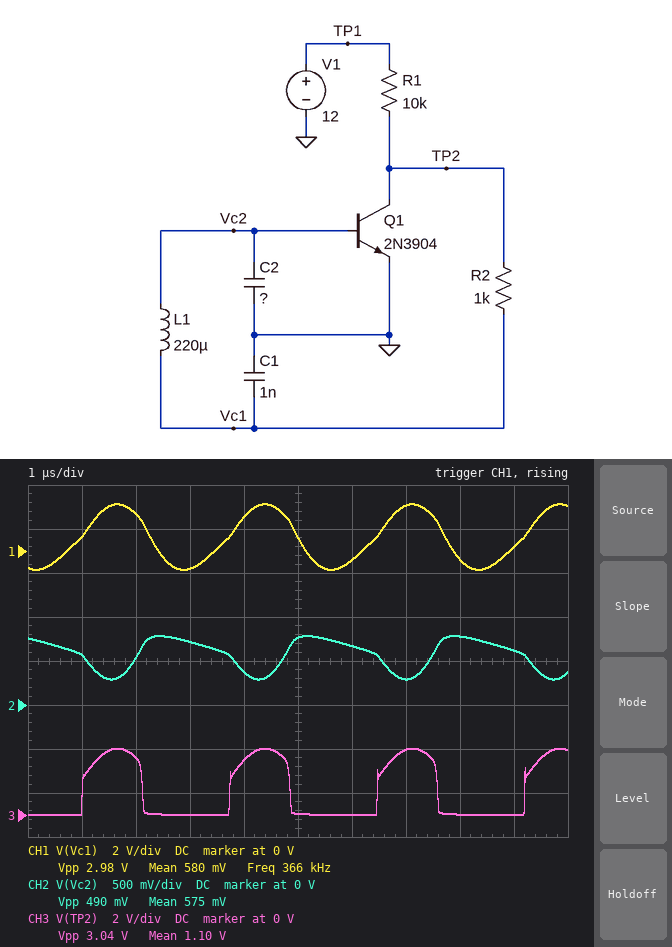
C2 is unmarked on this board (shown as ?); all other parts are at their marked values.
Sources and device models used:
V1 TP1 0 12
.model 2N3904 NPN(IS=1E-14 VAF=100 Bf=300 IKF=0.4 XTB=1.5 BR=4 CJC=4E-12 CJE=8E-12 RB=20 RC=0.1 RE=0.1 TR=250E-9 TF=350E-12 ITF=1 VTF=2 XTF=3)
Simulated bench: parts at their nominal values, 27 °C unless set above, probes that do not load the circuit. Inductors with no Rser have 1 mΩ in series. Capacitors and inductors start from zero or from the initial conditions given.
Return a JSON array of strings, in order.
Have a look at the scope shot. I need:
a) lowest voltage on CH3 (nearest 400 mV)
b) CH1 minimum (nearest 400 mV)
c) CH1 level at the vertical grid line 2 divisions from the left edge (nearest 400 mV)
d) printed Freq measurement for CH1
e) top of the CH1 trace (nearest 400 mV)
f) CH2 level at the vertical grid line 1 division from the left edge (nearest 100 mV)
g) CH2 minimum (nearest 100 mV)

["0 V", "-800 mV", "1.6 V", "366 kHz", "2.0 V", "600 mV", "300 mV"]
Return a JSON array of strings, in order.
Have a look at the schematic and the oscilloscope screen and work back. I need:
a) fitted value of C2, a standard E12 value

["3.3 nF"]
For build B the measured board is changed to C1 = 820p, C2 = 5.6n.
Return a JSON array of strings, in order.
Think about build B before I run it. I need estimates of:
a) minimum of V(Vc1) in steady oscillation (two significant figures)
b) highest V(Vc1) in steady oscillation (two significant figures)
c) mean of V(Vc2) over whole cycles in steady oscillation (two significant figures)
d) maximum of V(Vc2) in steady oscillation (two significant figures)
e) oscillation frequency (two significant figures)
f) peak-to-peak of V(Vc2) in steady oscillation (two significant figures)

["-940 mV", "2.3 V", "640 mV", "770 mV", "390 kHz", "290 mV"]
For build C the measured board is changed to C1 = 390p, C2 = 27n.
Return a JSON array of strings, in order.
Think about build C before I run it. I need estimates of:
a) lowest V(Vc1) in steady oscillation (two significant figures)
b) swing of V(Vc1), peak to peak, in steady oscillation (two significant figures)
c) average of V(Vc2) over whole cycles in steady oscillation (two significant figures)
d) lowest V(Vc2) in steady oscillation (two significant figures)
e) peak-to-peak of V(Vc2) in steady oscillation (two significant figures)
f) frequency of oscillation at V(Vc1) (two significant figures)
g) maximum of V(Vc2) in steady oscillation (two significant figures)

["-380 mV", "2.1 V", "660 mV", "650 mV", "30 mV", "510 kHz", "680 mV"]
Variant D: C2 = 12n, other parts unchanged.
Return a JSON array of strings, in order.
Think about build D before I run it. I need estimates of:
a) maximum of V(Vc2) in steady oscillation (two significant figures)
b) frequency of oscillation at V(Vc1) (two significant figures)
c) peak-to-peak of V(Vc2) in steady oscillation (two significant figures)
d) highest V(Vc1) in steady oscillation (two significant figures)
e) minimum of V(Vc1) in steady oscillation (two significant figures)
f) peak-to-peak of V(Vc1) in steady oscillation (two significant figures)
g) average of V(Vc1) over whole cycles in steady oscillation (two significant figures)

["760 mV", "340 kHz", "210 mV", "2.3 V", "-960 mV", "3.3 V", "660 mV"]
